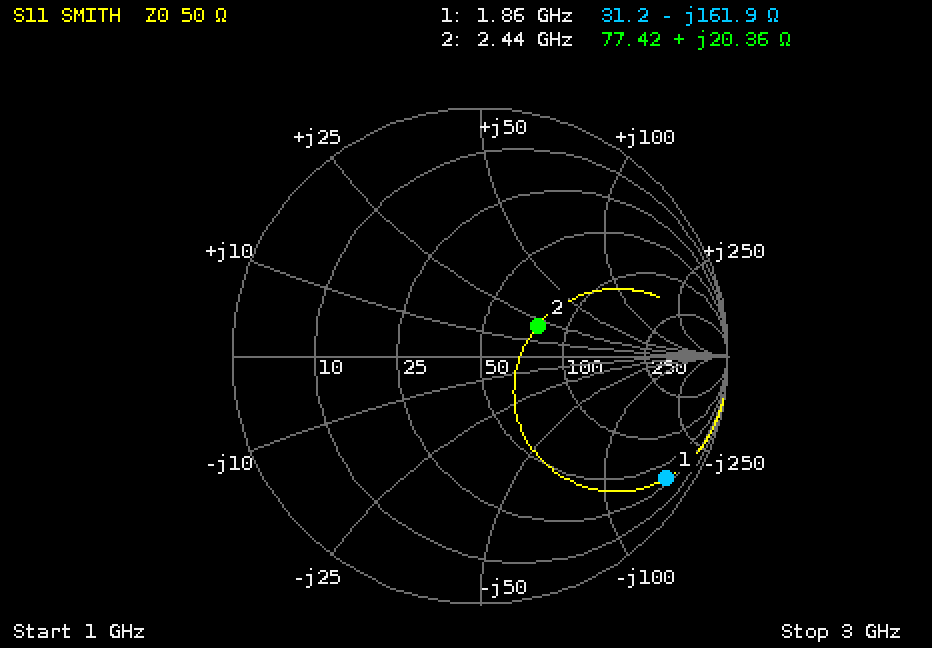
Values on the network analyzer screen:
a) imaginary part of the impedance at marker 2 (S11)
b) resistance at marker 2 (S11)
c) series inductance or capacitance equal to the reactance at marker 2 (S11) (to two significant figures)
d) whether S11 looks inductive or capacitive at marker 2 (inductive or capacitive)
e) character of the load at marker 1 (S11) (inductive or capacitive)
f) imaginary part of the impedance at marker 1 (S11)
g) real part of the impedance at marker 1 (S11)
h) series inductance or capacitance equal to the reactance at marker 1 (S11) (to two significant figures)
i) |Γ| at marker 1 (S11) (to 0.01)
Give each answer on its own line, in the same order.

+20.36 Ω
77.42 Ω
1.3 nH
inductive
capacitive
-161.9 Ω
31.2 Ω
530 fF
0.90
